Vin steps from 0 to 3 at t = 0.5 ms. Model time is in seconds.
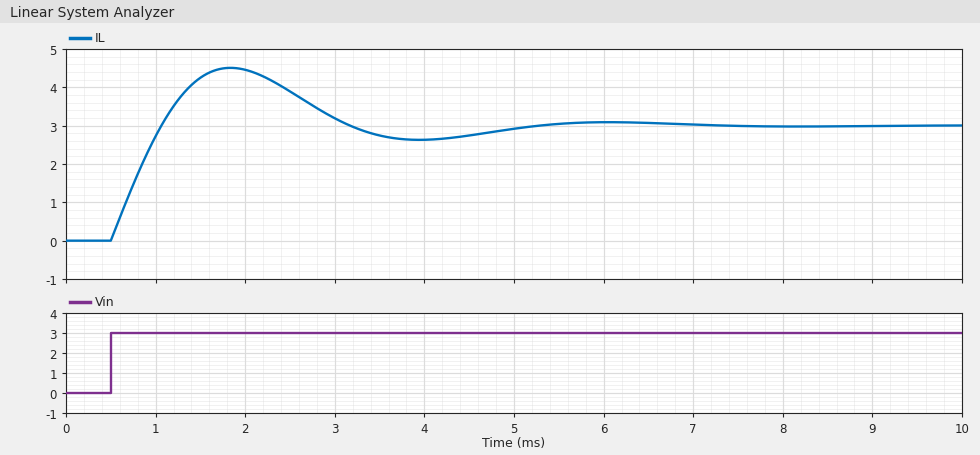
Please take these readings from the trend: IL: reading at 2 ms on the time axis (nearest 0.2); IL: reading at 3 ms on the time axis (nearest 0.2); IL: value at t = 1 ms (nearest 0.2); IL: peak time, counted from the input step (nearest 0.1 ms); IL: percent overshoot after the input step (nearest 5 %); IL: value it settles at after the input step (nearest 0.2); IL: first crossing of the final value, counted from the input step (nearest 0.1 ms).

4.4
3.2
2.8
1.3 ms
50 %
3.0
0.6 ms
